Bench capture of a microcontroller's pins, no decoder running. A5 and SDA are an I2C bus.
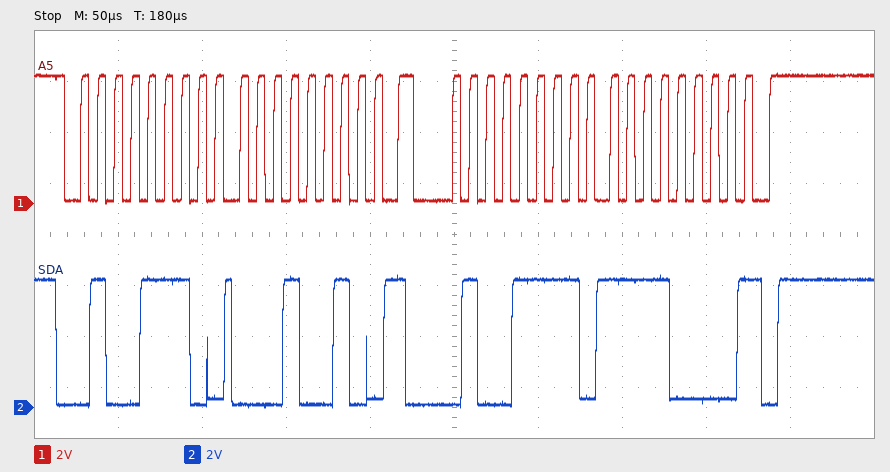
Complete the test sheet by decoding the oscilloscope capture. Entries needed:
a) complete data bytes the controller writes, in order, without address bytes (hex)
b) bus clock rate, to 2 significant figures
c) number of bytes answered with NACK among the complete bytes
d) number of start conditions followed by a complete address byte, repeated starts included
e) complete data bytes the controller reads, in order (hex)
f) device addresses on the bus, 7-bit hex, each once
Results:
12
100 kHz
1
2
F0
0x27
